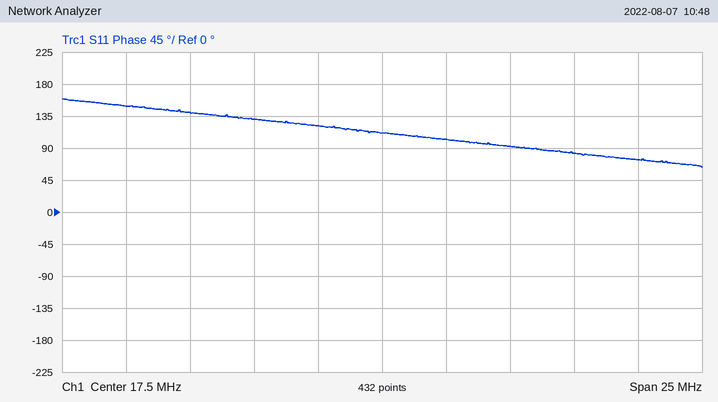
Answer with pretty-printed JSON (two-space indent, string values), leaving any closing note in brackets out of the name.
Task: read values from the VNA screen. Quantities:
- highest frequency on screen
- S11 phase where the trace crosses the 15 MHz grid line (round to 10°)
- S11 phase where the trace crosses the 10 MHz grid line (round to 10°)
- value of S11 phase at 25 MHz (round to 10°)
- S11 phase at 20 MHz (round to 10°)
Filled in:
{
  "highest frequency on screen": "30 MHz",
  "S11 phase where the trace crosses the 15 MHz grid line": "120°",
  "S11 phase where the trace crosses the 10 MHz grid line": "140°",
  "value of S11 phase at 25 MHz": "80°",
  "S11 phase at 20 MHz": "100°"
}
